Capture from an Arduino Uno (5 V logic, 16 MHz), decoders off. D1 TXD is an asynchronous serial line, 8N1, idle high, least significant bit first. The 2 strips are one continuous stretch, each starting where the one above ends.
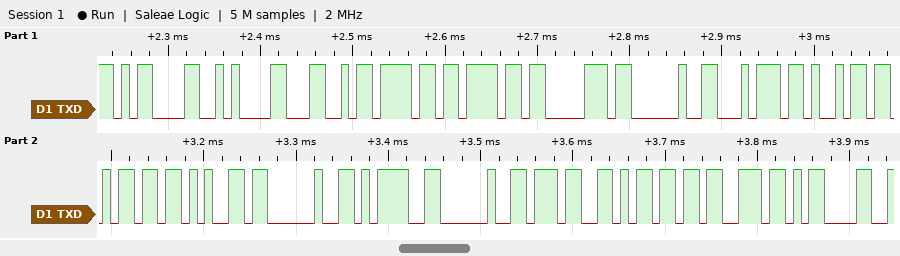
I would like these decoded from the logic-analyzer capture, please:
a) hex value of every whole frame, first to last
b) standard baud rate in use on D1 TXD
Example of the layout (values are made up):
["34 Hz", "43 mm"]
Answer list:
["0x0D 0x0A 0x4C 0x6F 0x6F 0x70 0x20 0x74 0x69 0x6D 0x65 0x20 0x3D 0x20 0x37 0x6D 0x73 0x0D", "115200 baud"]
